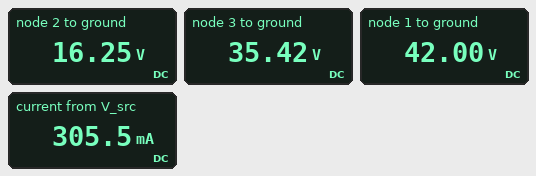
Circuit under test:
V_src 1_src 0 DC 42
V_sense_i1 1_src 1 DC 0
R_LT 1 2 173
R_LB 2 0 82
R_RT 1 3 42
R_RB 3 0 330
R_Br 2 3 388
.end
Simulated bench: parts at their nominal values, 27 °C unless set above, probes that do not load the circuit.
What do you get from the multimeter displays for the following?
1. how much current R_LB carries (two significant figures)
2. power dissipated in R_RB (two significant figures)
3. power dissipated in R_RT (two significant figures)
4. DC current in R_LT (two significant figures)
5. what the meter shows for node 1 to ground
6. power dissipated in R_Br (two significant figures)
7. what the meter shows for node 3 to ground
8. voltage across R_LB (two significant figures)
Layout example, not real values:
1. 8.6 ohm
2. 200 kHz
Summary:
1. 200 mA
2. 3.8 W
3. 1.0 W
4. 150 mA
5. 42.00 V
6. 950 mW
7. 35.42 V
8. 16 V
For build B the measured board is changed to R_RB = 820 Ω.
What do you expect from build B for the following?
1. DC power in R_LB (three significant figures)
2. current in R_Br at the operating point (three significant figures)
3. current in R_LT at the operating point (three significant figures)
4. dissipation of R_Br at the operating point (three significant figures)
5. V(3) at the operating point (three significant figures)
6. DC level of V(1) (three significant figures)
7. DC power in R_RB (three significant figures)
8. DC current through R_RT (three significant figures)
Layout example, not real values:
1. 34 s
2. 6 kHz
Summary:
1. 3.34 W
2. 54.7 mA
3. 147 mA
4. 1.16 W
5. 37.8 V
6. 42.0 V
7. 1.74 W
8. 101 mA
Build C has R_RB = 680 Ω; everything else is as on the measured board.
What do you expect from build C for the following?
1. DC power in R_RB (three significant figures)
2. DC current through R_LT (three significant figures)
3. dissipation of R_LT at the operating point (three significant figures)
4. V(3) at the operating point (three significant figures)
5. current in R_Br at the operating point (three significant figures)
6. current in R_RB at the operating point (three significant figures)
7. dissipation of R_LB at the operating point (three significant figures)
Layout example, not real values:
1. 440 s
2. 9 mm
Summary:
1. 2.06 W
2. 147 mA
3. 3.76 W
4. 37.4 V
5. 53.9 mA
6. 55.0 mA
7. 3.32 W
